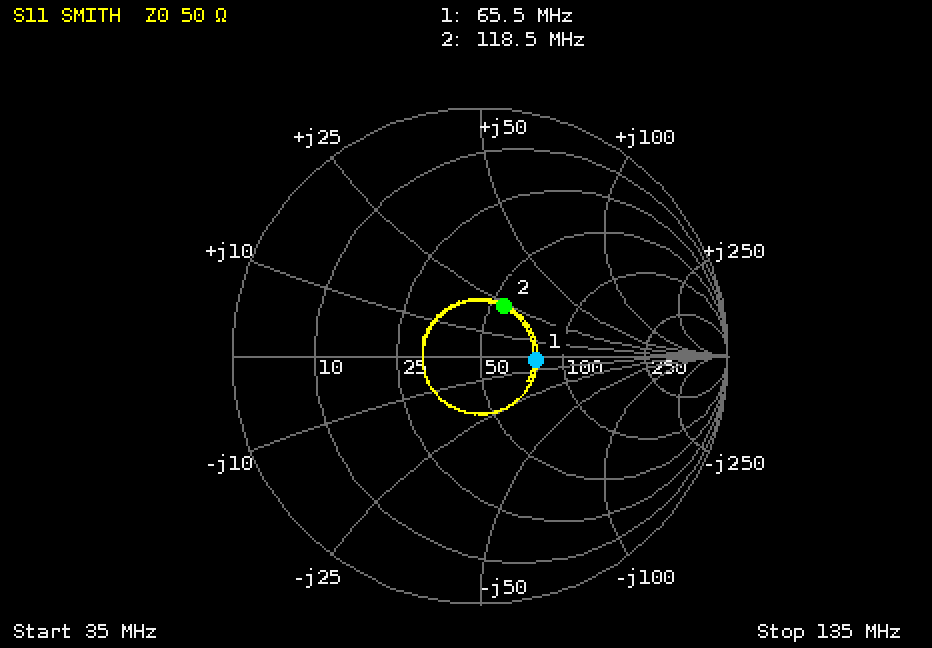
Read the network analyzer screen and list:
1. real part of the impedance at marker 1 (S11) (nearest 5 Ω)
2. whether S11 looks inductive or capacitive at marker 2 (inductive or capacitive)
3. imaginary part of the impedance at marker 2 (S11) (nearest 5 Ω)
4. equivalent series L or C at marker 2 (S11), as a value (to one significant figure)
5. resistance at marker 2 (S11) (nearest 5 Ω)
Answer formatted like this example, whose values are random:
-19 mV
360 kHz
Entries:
80 Ω
inductive
+25 Ω
30 nH
55 Ω
